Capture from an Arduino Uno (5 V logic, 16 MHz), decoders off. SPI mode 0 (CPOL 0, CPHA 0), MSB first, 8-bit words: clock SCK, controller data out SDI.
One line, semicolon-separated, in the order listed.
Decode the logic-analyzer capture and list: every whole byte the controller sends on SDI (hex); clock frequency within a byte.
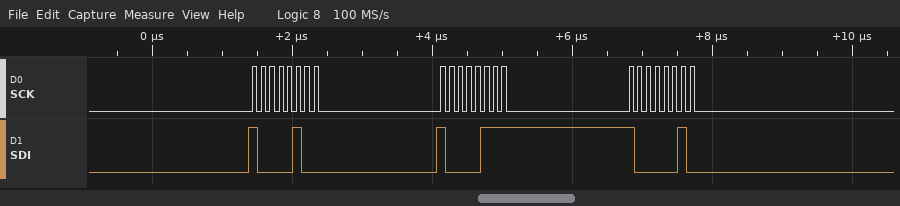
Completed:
84 87 82; 8 MHz
